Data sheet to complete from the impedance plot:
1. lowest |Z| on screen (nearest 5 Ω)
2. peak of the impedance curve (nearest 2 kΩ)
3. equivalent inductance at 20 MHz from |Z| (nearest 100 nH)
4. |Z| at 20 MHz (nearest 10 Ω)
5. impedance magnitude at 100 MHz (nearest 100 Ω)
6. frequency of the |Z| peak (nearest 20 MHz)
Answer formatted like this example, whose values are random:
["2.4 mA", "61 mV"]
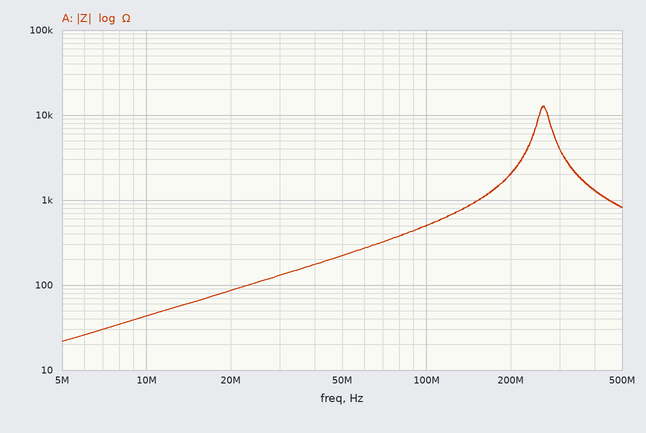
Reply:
["20 Ω", "12 kΩ", "700 nH", "90 Ω", "500 Ω", "260 MHz"]
